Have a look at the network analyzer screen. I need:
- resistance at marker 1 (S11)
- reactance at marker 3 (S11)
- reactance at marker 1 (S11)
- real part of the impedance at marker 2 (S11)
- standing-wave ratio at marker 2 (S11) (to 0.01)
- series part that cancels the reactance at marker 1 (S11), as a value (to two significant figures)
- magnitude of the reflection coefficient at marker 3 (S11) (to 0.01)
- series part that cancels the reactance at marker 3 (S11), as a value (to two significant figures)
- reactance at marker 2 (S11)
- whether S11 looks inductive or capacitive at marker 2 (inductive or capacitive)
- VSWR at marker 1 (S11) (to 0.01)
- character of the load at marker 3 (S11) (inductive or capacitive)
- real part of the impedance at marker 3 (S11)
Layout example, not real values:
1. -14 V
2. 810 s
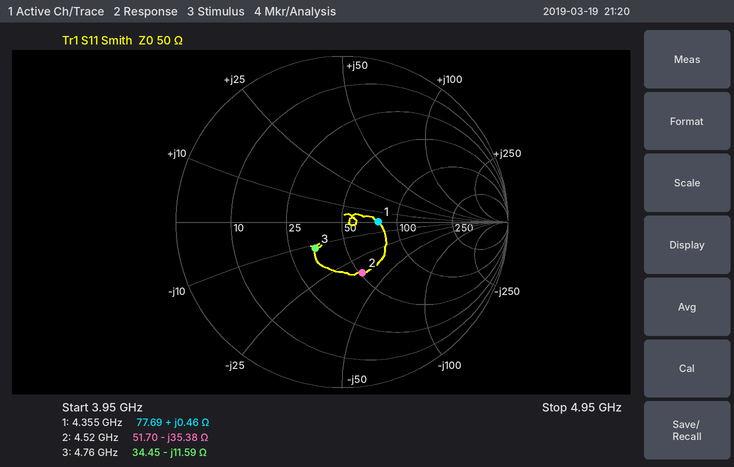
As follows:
1. 77.69 Ω
2. -11.59 Ω
3. +0.46 Ω
4. 51.70 Ω
5. 1.98
6. 79 pF
7. 0.23
8. 390 pH
9. -35.38 Ω
10. capacitive
11. 1.55
12. capacitive
13. 34.45 Ω
